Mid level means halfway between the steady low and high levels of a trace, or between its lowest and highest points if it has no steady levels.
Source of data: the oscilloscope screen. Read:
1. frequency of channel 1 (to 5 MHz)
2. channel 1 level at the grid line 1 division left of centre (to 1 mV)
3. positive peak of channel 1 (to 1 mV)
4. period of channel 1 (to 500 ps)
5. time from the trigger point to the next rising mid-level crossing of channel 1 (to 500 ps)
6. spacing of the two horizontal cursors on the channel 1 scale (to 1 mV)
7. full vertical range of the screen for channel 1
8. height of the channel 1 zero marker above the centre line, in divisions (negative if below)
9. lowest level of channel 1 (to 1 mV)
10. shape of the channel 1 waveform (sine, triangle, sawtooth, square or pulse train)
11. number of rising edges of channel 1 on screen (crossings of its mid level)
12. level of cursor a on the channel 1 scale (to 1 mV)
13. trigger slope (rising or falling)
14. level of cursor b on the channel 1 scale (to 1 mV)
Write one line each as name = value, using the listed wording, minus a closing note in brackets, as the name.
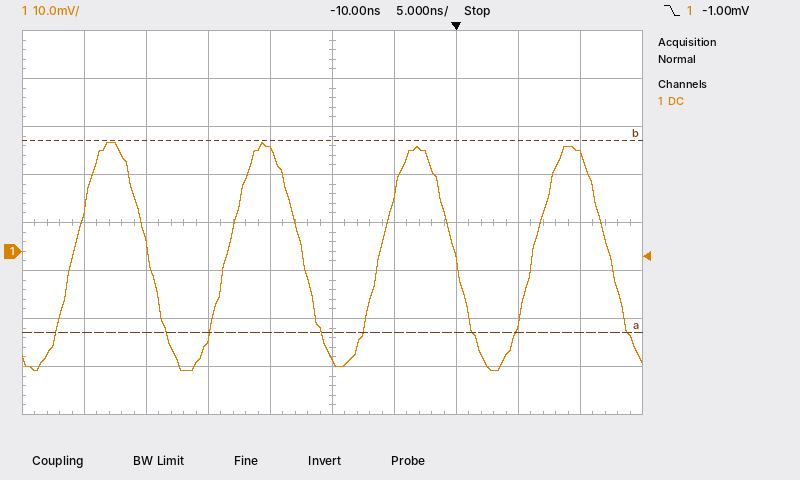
frequency of channel 1 = 80 MHz
channel 1 level at the grid line 1 division left of centre = 21 mV
positive peak of channel 1 = 23 mV
period of channel 1 = 12.5 ns
time from the trigger point to the next rising mid-level crossing of channel 1 = 6.0 ns
spacing of the two horizontal cursors on the channel 1 scale = 40 mV
full vertical range of the screen for channel 1 = 80 mV
height of the channel 1 zero marker above the centre line, in divisions = -0.6 div
lowest level of channel 1 = -25 mV
shape of the channel 1 waveform = sine
number of rising edges of channel 1 on screen = 4
level of cursor a on the channel 1 scale = -17 mV
trigger slope = falling
level of cursor b on the channel 1 scale = 23 mV
